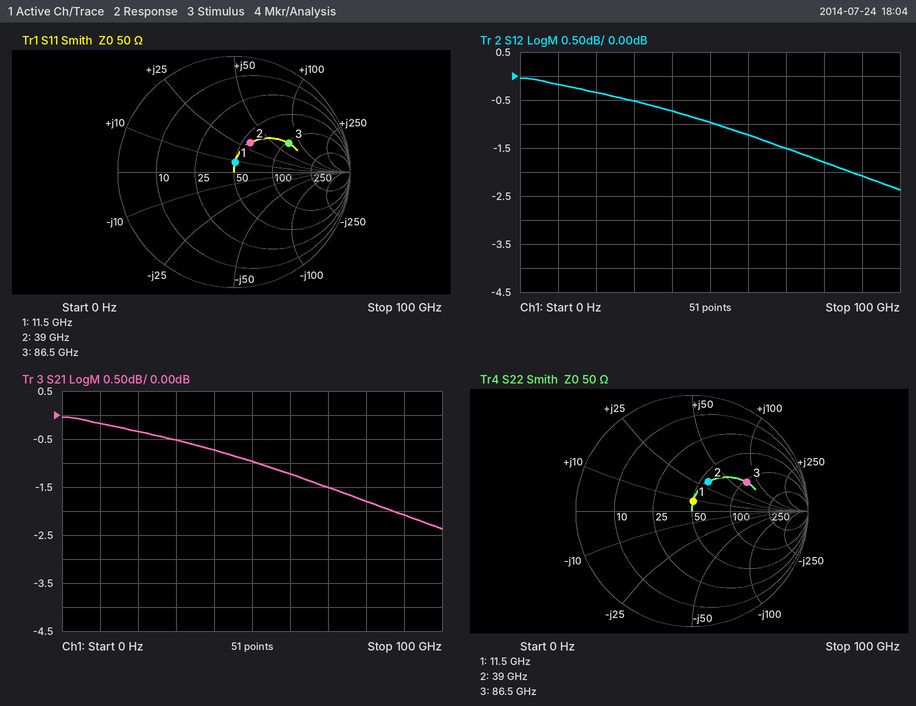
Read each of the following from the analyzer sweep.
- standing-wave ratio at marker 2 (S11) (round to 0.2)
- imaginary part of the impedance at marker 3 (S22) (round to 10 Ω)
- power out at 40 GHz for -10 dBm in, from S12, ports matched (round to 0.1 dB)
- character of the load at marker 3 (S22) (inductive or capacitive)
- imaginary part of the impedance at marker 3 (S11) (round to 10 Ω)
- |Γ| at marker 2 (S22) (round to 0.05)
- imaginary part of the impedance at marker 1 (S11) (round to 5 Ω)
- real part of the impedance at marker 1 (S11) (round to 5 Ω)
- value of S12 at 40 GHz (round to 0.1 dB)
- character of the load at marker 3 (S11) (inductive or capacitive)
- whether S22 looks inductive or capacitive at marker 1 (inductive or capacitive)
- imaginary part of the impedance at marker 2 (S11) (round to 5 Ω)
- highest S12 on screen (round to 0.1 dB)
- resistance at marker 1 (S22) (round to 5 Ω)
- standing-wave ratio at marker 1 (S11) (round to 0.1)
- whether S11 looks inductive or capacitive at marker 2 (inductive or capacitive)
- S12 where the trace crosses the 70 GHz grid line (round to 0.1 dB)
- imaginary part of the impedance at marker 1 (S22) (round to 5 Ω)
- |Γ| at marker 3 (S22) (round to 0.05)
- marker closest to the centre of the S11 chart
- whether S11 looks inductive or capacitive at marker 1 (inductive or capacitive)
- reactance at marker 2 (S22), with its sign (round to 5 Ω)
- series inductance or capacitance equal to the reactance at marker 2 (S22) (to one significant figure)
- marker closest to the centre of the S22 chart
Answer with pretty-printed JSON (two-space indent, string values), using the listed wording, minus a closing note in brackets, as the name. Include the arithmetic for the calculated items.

{
  "standing-wave ratio at marker 2 (S11)": "1.8",
  "imaginary part of the impedance at marker 3 (S22)": "+70 Ω",
  "power out at 40 GHz for -10 dBm in, from S12, ports matched": "-10 dBm + (-0.7 dB) = -10.7 dBm",
  "character of the load at marker 3 (S22)": "inductive",
  "imaginary part of the impedance at marker 3 (S11)": "+70 Ω",
  "|Γ| at marker 2 (S22)": "0.30",
  "imaginary part of the impedance at marker 1 (S11)": "+10 Ω",
  "real part of the impedance at marker 1 (S11)": "50 Ω",
  "value of S12 at 40 GHz": "-0.7 dB",
  "character of the load at marker 3 (S11)": "inductive",
  "whether S22 looks inductive or capacitive at marker 1": "inductive",
  "imaginary part of the impedance at marker 2 (S11)": "+30 Ω",
  "highest S12 on screen": "0.0 dB",
  "resistance at marker 1 (S22)": "50 Ω",
  "standing-wave ratio at marker 1 (S11)": "1.2",
  "whether S11 looks inductive or capacitive at marker 2": "inductive",
  "S12 where the trace crosses the 70 GHz grid line": "-1.5 dB",
  "imaginary part of the impedance at marker 1 (S22)": "+10 Ω",
  "|Γ| at marker 3 (S22)": "0.55",
  "marker closest to the centre of the S11 chart": "marker 1",
  "whether S11 looks inductive or capacitive at marker 1": "inductive",
  "reactance at marker 2 (S22), with its sign": "+30 Ω",
  "series inductance or capacitance equal to the reactance at marker 2 (S22)": "L = 30 Ω/(2π × 39 GHz) ≈ 122 pH, so 100 pH to one significant figure",
  "marker closest to the centre of the S22 chart": "marker 1"
}
